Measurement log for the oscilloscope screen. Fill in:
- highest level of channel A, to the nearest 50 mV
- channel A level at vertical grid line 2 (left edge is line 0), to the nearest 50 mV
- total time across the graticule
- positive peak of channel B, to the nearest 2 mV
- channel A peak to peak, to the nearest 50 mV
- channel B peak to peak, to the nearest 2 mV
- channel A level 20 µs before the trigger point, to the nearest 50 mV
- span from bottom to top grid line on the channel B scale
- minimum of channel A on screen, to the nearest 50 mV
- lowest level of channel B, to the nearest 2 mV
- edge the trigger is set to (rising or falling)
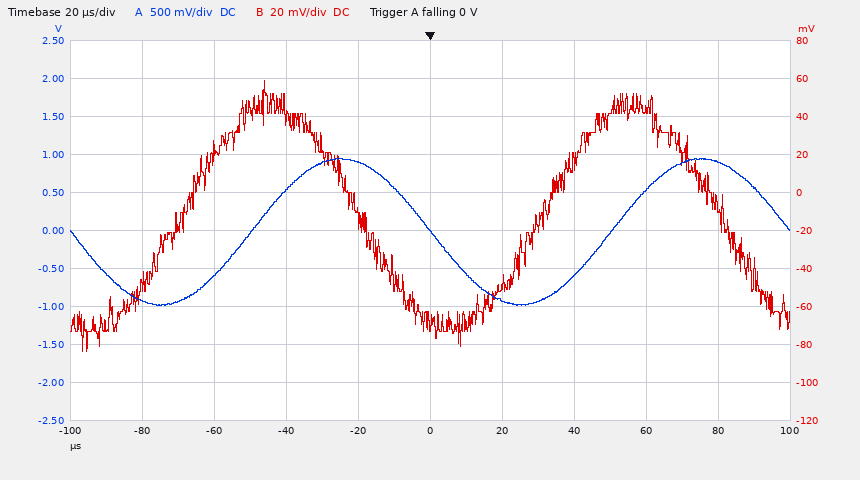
950 mV
-600 mV
200 µs
58 mV
1.95 V
142 mV
900 mV
200 mV
-1.00 V
-84 mV
falling
